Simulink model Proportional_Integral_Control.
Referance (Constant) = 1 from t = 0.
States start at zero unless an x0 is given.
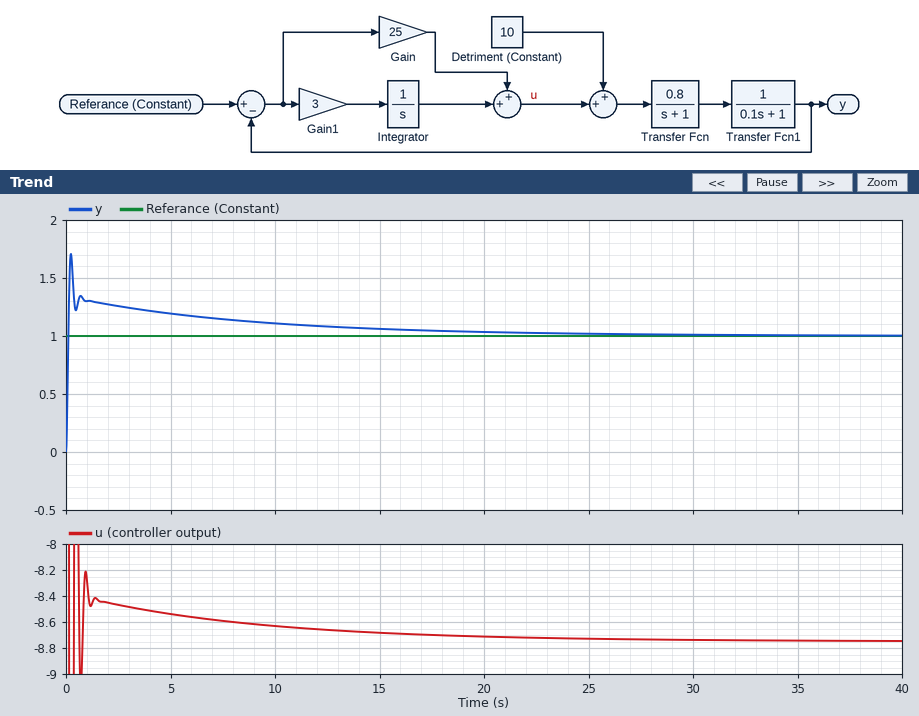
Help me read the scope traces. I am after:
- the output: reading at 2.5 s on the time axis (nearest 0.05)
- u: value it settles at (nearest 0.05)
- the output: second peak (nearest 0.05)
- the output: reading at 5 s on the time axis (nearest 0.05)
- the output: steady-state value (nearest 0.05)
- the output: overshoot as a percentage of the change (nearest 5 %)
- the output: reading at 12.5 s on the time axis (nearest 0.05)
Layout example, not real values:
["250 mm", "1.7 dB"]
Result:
["1.25", "-8.75", "1.35", "1.20", "1.00", "70 %", "1.10"]
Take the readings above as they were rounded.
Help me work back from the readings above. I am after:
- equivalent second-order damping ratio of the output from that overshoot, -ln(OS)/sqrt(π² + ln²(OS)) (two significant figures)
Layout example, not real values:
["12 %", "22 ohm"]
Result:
["0.11"]
